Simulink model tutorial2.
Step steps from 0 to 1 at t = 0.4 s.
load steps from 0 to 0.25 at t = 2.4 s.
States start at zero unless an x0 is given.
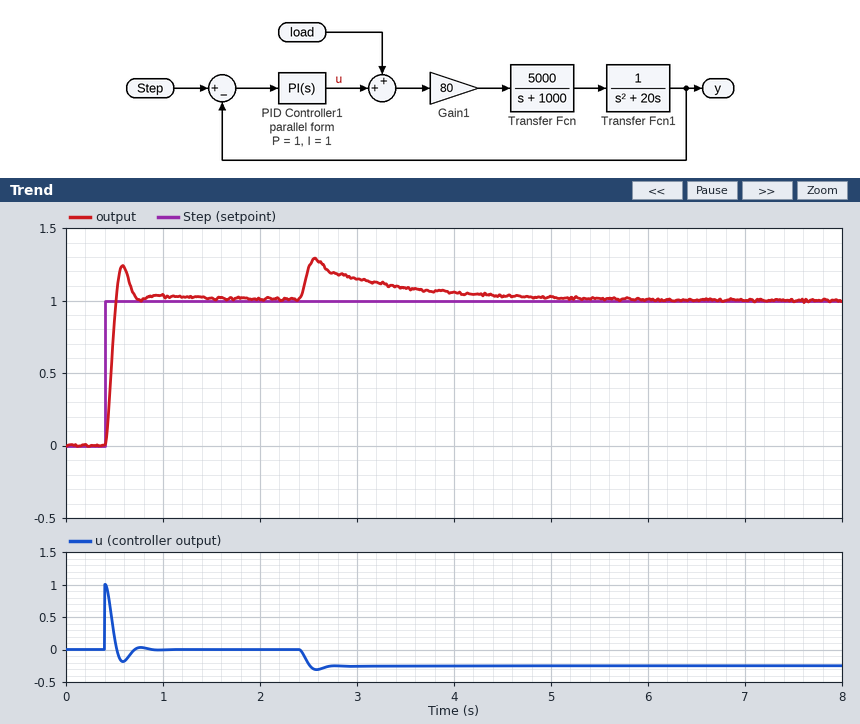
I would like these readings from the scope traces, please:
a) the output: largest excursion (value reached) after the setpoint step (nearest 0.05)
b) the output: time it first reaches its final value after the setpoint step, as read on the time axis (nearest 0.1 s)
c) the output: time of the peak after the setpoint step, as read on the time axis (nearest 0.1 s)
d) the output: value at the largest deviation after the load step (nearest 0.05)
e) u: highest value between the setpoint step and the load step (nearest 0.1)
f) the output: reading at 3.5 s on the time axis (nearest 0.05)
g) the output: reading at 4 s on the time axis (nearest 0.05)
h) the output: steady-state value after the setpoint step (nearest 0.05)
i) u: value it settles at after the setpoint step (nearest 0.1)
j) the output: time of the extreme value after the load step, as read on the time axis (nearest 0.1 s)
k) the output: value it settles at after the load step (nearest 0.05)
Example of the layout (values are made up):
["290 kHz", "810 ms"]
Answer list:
["1.25", "0.5 s", "0.6 s", "1.30", "1.0", "1.10", "1.05", "1.00", "0.0", "2.6 s", "1.00"]
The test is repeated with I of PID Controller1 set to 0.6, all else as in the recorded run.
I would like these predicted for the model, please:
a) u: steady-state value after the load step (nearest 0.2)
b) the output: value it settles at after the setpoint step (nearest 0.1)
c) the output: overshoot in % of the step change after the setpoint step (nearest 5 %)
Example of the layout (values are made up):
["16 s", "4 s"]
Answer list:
["-0.2", "1.0", "20 %"]
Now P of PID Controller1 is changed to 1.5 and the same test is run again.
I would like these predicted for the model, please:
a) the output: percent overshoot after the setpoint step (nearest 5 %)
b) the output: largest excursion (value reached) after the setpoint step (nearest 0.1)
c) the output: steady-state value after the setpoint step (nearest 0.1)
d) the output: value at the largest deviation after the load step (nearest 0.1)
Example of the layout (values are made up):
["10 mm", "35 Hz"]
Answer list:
["30 %", "1.3", "1.0", "1.2"]
